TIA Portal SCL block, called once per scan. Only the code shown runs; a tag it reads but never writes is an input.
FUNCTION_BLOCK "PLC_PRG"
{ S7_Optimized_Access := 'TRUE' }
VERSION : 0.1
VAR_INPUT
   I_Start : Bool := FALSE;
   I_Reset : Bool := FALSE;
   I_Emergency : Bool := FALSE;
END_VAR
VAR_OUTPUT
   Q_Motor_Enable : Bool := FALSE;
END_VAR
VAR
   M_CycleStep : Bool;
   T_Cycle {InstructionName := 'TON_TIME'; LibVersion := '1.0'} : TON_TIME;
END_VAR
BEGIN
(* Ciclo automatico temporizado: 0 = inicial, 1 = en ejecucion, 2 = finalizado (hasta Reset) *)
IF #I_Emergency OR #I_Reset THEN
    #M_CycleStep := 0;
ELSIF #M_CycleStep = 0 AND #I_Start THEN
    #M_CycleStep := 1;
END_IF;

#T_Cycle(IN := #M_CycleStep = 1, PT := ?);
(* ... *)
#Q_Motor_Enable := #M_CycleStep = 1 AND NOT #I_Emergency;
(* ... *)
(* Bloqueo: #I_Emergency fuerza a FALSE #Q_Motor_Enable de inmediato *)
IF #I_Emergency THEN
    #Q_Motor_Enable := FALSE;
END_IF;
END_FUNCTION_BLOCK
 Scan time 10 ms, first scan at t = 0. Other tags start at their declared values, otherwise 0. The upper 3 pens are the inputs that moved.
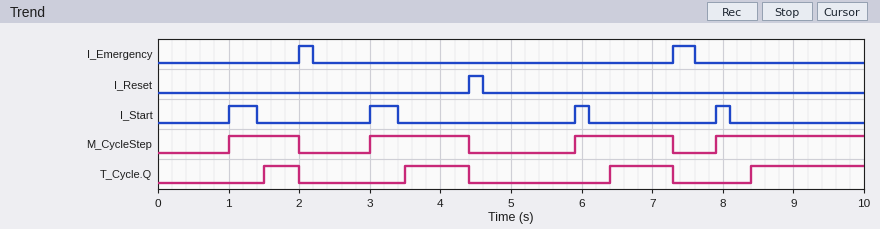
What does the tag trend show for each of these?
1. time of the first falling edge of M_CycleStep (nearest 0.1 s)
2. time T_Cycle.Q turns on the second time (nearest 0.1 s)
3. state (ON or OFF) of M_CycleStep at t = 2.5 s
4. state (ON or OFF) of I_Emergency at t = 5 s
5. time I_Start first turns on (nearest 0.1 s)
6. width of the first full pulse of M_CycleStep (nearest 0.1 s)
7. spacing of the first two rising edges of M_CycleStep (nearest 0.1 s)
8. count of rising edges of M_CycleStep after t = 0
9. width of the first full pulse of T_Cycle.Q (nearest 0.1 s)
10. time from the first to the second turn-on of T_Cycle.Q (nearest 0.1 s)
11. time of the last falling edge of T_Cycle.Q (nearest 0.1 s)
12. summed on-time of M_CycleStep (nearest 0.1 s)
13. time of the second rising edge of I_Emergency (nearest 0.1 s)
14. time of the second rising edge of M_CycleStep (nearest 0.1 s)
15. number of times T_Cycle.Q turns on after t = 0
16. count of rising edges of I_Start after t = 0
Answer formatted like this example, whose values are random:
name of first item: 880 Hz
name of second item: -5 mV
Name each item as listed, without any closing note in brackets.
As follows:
time of the first falling edge of M_CycleStep: 2.0 s
time T_Cycle.Q turns on the second time: 3.5 s
state (ON or OFF) of M_CycleStep at t = 2.5 s: OFF
state (ON or OFF) of I_Emergency at t = 5 s: OFF
time I_Start first turns on: 1.0 s
width of the first full pulse of M_CycleStep: 1.0 s
spacing of the first two rising edges of M_CycleStep: 2.0 s
count of rising edges of M_CycleStep after t = 0: 4
width of the first full pulse of T_Cycle.Q: 0.5 s
time from the first to the second turn-on of T_Cycle.Q: 2.0 s
time of the last falling edge of T_Cycle.Q: 7.3 s
summed on-time of M_CycleStep: 5.9 s
time of the second rising edge of I_Emergency: 7.3 s
time of the second rising edge of M_CycleStep: 3.0 s
number of times T_Cycle.Q turns on after t = 0: 4
count of rising edges of I_Start after t = 0: 4
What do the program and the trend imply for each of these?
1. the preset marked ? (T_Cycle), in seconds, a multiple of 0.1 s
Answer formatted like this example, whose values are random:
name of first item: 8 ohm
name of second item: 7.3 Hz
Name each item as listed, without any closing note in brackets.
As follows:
the preset marked ? (T_Cycle), in seconds, a multiple of 0.1 s: 0.5 s
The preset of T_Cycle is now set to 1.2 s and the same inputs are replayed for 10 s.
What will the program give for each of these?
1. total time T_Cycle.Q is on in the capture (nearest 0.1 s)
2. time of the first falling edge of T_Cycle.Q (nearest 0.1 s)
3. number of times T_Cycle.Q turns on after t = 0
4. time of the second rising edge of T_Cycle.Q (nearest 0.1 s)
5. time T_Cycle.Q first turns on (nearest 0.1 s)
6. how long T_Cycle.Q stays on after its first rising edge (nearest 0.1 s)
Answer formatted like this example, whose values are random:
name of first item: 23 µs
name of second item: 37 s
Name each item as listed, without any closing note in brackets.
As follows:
total time T_Cycle.Q is on in the capture: 1.3 s
time of the first falling edge of T_Cycle.Q: 4.4 s
number of times T_Cycle.Q turns on after t = 0: 3
time of the second rising edge of T_Cycle.Q: 7.1 s
time T_Cycle.Q first turns on: 4.2 s
how long T_Cycle.Q stays on after its first rising edge: 0.2 s
